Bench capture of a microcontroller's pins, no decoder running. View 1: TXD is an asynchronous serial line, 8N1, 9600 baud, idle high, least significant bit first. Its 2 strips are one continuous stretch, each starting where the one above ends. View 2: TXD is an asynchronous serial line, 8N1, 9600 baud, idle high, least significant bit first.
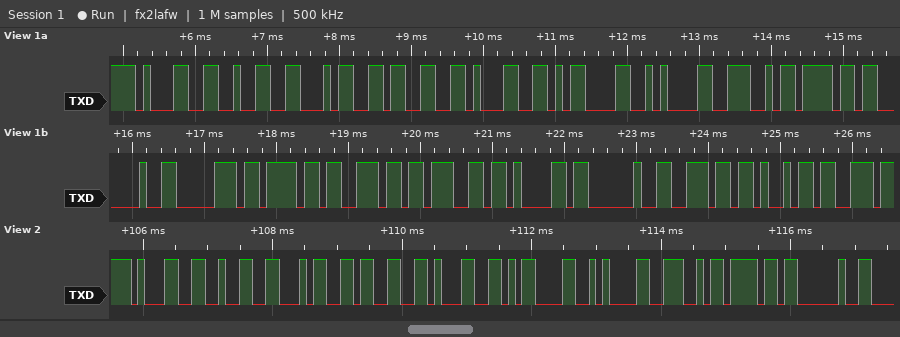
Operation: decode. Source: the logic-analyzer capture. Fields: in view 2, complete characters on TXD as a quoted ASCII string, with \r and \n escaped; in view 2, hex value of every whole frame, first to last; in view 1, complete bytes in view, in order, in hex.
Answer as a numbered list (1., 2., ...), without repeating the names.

1. "12431\r\nNo "
2. 31 32 34 33 31 0D 0A 4E 6F 20
3. 31 32 34 33 31 0D 0A 4E 6F 20 70 6F 6E 67 61 20 6E 69
